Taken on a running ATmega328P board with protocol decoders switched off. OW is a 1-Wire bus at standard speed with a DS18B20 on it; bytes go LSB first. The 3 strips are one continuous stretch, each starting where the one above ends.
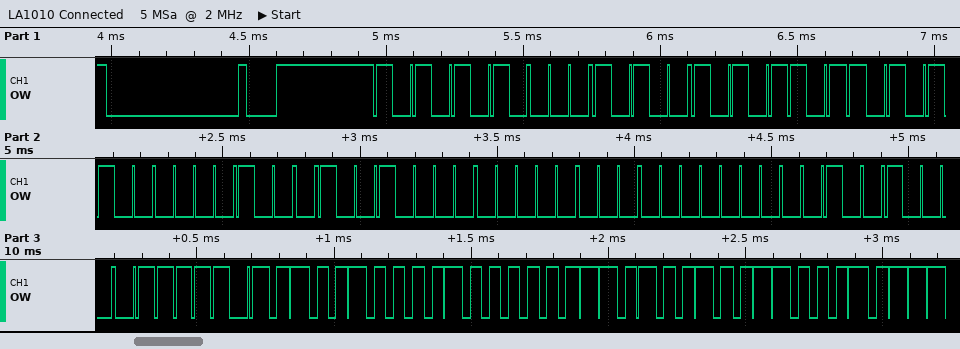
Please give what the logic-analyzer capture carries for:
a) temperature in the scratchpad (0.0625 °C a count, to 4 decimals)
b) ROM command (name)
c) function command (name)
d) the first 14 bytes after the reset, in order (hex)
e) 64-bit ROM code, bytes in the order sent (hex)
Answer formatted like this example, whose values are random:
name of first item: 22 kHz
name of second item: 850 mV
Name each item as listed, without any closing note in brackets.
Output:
temperature in the scratchpad: 33.1250 °C
ROM command: Match ROM
function command: Read Scratchpad
the first 14 bytes after the reset, in order: 55 28 B5 35 10 09 00 00 12 BE 12 02 4B 46
64-bit ROM code, bytes in the order sent: 28 B5 35 10 09 00 00 12
